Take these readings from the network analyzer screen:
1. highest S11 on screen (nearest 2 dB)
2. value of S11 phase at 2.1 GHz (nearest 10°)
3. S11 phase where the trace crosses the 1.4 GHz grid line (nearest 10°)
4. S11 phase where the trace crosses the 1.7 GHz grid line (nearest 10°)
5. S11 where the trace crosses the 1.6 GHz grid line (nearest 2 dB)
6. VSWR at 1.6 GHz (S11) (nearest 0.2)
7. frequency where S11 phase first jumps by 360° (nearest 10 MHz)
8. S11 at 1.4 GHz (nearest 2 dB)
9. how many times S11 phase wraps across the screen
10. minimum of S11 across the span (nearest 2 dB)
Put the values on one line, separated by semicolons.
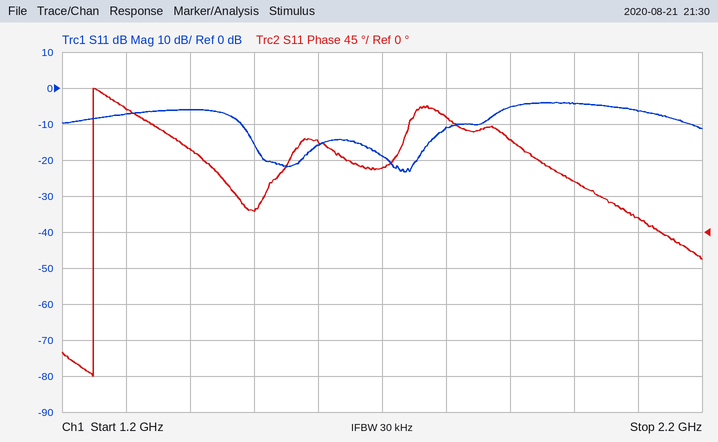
-4 dB; 20°; 100°; 80°; -16 dB; 1.4; 1.25 GHz; -6 dB; 1; -24 dB
